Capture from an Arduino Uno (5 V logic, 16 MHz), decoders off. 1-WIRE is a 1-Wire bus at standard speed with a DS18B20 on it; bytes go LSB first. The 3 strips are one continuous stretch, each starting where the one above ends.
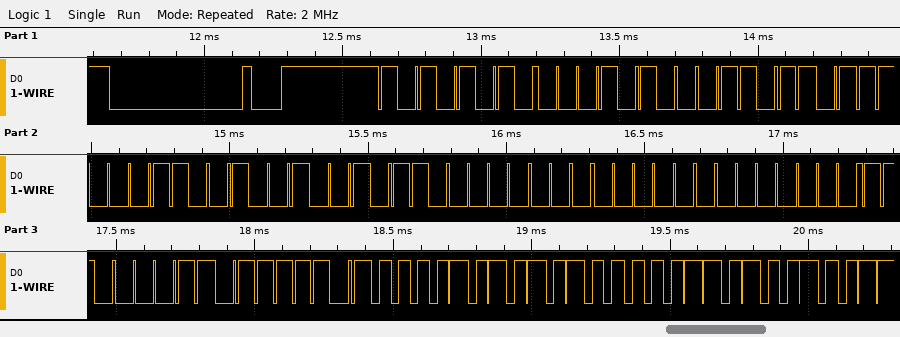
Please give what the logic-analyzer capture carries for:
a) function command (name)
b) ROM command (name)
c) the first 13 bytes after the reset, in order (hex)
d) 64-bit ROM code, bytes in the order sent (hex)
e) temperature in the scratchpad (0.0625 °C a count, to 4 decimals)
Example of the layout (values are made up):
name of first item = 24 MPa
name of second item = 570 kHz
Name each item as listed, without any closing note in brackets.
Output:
function command = Read Scratchpad
ROM command = Match ROM
the first 13 bytes after the reset, in order = 55 28 B6 63 92 06 00 00 C3 BE 50 05 4B
64-bit ROM code, bytes in the order sent = 28 B6 63 92 06 00 00 C3
temperature in the scratchpad = 85.0000 °C
